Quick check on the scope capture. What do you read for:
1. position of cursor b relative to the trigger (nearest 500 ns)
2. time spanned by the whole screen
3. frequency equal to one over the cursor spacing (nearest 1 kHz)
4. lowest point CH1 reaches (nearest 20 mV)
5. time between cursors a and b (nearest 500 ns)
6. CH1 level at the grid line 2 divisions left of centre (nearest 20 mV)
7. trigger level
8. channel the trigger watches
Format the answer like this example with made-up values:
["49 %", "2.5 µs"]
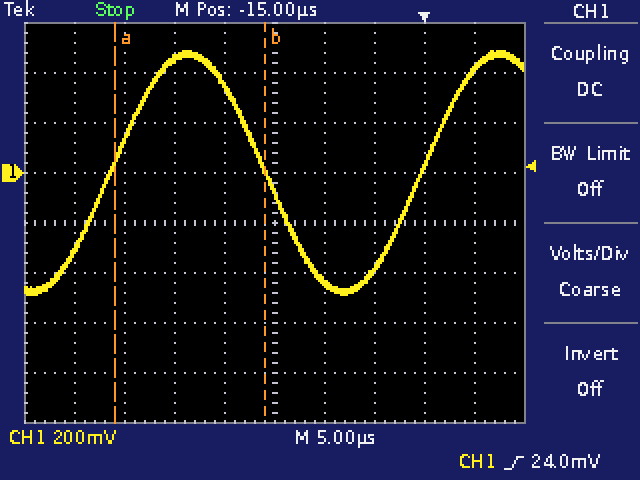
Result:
["-16.0 µs", "50 µs", "67 kHz", "-480 mV", "15.0 µs", "460 mV", "24.0 mV", "CH1"]
